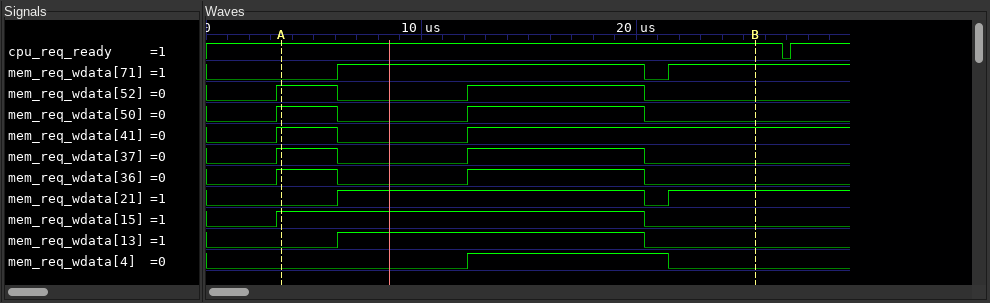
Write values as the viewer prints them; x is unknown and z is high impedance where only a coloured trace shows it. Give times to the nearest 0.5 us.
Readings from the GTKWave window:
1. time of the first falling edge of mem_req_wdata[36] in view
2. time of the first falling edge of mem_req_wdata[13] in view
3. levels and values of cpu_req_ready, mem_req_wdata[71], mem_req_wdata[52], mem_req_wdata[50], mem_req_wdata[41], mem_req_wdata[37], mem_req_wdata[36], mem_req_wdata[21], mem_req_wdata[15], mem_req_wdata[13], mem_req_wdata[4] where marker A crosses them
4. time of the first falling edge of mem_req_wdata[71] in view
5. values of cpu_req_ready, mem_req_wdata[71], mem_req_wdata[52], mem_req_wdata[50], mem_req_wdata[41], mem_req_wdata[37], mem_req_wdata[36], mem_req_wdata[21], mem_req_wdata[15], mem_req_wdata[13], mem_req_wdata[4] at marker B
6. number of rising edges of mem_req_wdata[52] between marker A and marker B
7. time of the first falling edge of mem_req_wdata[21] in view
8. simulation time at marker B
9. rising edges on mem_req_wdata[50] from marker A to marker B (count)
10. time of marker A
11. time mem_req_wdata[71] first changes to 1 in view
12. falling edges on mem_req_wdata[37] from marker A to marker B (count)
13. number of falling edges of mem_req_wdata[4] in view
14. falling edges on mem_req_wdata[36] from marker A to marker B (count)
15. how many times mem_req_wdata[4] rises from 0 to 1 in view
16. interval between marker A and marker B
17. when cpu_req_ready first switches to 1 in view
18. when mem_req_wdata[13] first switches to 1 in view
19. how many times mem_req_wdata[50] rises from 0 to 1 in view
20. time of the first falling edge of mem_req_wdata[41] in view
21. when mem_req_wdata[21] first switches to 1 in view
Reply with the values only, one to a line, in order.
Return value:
6 us
20.5 us
cpu_req_ready=1, mem_req_wdata[71]=0, mem_req_wdata[52]=1, mem_req_wdata[50]=1, mem_req_wdata[41]=1, mem_req_wdata[37]=1, mem_req_wdata[36]=1, mem_req_wdata[21]=0, mem_req_wdata[15]=1, mem_req_wdata[13]=0, mem_req_wdata[4]=0
20.5 us
cpu_req_ready=1, mem_req_wdata[71]=1, mem_req_wdata[52]=0, mem_req_wdata[50]=0, mem_req_wdata[41]=1, mem_req_wdata[37]=0, mem_req_wdata[36]=0, mem_req_wdata[21]=1, mem_req_wdata[15]=0, mem_req_wdata[13]=0, mem_req_wdata[4]=0
1
20.5 us
25.5 us
1
3.5 us
6 us
2
1
2
1
22 us
27 us
6 us
2
6 us
6 us
